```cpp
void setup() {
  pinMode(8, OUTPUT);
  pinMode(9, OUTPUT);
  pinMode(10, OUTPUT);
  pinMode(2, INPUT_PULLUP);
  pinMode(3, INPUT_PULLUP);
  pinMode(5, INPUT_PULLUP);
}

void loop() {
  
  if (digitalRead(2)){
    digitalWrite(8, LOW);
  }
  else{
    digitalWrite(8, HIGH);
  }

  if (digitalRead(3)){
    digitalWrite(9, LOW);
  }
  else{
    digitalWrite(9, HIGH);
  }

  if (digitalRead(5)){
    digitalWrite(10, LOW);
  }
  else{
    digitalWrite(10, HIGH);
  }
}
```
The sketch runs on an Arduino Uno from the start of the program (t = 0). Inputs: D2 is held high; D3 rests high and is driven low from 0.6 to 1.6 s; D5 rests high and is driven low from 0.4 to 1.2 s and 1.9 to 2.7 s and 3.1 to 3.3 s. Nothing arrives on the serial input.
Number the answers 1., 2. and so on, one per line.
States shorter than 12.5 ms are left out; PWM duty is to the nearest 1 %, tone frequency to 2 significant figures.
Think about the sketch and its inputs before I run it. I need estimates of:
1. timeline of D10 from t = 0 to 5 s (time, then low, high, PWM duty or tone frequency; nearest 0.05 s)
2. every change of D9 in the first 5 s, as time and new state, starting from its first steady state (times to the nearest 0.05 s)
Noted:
1. 0 s low; 0.4 s high; 1.2 s low; 1.9 s high; 2.7 s low; 3.1 s high; 3.3 s low
2. 0 s low; 0.6 s high; 1.6 s low
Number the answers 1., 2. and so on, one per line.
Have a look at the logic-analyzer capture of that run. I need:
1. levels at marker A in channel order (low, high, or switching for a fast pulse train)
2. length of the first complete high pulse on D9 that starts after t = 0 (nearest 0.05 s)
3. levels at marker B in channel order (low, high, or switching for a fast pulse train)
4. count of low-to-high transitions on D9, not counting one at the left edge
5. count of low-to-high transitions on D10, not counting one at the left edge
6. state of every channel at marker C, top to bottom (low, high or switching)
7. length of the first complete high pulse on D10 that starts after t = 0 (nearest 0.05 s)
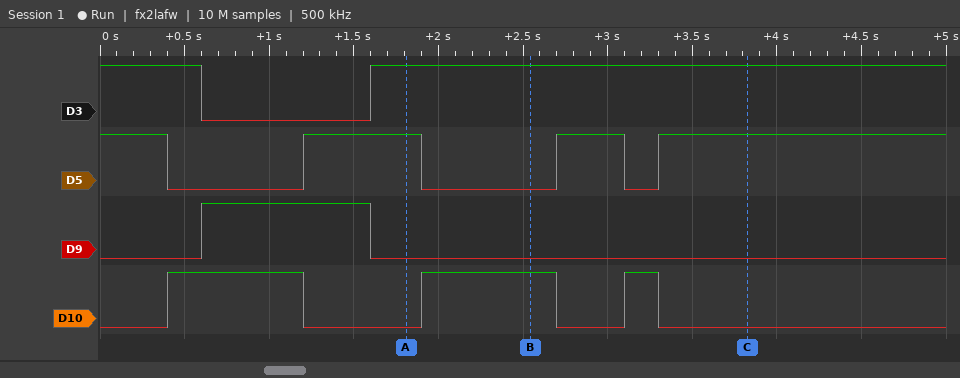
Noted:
1. D3 high, D5 high, D9 low, D10 low
2. 1.00 s
3. D3 high, D5 low, D9 low, D10 high
4. 1
5. 3
6. D3 high, D5 high, D9 low, D10 low
7. 0.80 s
